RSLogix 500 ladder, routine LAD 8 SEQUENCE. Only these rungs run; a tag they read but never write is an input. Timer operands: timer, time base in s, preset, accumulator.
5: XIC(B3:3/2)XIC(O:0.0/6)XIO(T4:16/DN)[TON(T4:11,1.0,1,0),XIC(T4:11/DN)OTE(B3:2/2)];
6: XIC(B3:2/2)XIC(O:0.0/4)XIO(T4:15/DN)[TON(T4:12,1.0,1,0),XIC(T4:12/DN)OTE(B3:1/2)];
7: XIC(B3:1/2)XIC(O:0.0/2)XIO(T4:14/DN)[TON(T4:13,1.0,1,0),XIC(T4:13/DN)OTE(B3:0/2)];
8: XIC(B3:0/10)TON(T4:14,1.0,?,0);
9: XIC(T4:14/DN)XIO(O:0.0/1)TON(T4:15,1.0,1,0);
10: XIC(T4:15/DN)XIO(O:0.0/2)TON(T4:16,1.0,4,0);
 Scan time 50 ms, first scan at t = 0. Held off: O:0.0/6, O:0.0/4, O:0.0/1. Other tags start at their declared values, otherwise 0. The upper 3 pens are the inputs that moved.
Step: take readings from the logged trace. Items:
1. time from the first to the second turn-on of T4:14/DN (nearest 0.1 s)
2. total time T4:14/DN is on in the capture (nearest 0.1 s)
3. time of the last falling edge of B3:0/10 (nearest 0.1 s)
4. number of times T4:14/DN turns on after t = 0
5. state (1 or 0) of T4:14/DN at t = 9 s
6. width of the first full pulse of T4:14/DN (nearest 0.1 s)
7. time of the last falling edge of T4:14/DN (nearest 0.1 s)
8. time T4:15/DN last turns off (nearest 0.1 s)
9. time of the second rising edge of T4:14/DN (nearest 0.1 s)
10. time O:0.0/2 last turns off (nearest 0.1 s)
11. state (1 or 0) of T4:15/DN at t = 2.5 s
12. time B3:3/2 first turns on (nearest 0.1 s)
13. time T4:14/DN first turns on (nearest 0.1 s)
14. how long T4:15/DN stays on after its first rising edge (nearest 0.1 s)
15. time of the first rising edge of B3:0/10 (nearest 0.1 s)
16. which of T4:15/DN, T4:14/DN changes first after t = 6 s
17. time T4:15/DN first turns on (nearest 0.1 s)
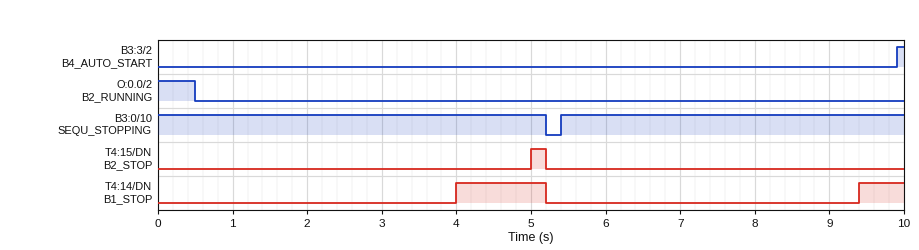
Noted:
5.4 s
1.8 s
5.2 s
2
0
1.2 s
5.2 s
5.2 s
9.4 s
0.5 s
0
9.9 s
4.0 s
0.2 s
5.4 s
T4:14/DN
5.0 s
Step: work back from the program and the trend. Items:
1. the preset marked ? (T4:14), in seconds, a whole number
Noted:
4 s
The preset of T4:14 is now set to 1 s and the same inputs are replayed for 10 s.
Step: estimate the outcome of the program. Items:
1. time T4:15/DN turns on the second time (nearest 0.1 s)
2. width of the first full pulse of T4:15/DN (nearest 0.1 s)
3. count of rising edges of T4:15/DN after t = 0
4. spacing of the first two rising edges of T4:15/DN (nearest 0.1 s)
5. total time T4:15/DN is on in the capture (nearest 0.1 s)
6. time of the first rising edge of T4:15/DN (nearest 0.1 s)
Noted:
7.4 s
3.2 s
2
5.4 s
5.8 s
2.0 s
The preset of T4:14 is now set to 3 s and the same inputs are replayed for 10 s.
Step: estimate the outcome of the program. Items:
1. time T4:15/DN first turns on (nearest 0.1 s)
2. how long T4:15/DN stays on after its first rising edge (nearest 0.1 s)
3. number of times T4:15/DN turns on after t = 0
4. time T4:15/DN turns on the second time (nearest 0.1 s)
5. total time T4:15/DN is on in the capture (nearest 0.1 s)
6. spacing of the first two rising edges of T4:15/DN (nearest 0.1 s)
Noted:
4.0 s
1.2 s
2
9.4 s
1.8 s
5.4 s
